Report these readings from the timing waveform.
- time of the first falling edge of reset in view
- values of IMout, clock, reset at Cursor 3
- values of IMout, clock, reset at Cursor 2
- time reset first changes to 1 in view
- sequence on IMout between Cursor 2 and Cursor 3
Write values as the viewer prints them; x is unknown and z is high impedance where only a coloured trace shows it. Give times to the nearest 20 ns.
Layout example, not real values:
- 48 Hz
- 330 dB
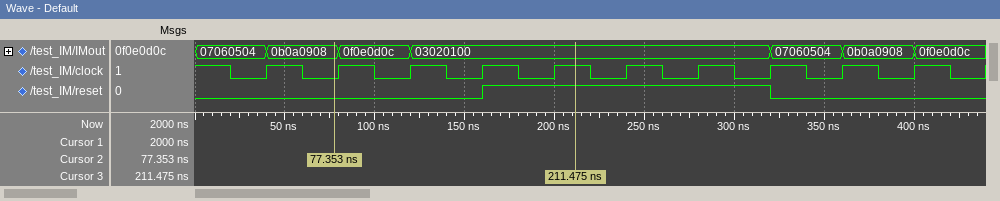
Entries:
- 320 ns
- IMout=03020100, clock=1, reset=1
- IMout=0b0a0908, clock=0, reset=0
- 160 ns
- 0b0a0908, 0f0e0d0c, 03020100
